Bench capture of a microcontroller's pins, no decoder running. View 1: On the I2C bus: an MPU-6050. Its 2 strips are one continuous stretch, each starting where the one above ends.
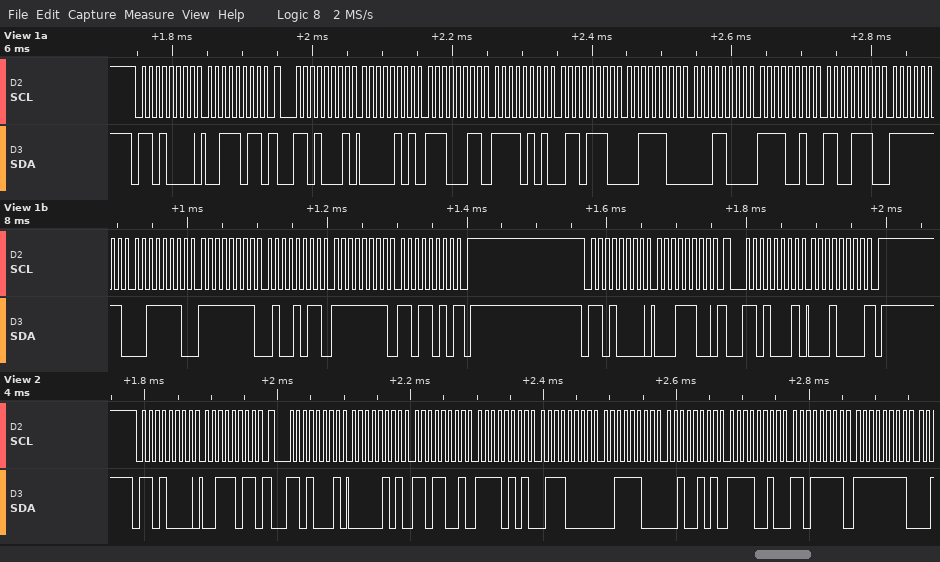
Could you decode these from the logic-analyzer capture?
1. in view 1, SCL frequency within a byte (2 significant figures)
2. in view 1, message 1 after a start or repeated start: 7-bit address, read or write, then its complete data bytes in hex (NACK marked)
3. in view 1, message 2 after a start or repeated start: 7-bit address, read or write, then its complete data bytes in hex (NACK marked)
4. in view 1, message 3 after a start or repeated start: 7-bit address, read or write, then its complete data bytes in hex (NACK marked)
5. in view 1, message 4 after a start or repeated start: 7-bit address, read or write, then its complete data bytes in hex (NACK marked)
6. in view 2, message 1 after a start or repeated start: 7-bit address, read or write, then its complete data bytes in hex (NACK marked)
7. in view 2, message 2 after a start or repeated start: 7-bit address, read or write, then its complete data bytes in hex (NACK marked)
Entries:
100 kHz
0x68 write: 3B
0x68 read: 05 E3 F5 6E 3C 18 F2 CE FF 3E FF 4B FF DA NACK
0x68 write: 1C
0x68 read: 10 NACK
0x68 write: 3B
0x68 read: 05 D9 F5 70 3C 25 F2 DF FF
